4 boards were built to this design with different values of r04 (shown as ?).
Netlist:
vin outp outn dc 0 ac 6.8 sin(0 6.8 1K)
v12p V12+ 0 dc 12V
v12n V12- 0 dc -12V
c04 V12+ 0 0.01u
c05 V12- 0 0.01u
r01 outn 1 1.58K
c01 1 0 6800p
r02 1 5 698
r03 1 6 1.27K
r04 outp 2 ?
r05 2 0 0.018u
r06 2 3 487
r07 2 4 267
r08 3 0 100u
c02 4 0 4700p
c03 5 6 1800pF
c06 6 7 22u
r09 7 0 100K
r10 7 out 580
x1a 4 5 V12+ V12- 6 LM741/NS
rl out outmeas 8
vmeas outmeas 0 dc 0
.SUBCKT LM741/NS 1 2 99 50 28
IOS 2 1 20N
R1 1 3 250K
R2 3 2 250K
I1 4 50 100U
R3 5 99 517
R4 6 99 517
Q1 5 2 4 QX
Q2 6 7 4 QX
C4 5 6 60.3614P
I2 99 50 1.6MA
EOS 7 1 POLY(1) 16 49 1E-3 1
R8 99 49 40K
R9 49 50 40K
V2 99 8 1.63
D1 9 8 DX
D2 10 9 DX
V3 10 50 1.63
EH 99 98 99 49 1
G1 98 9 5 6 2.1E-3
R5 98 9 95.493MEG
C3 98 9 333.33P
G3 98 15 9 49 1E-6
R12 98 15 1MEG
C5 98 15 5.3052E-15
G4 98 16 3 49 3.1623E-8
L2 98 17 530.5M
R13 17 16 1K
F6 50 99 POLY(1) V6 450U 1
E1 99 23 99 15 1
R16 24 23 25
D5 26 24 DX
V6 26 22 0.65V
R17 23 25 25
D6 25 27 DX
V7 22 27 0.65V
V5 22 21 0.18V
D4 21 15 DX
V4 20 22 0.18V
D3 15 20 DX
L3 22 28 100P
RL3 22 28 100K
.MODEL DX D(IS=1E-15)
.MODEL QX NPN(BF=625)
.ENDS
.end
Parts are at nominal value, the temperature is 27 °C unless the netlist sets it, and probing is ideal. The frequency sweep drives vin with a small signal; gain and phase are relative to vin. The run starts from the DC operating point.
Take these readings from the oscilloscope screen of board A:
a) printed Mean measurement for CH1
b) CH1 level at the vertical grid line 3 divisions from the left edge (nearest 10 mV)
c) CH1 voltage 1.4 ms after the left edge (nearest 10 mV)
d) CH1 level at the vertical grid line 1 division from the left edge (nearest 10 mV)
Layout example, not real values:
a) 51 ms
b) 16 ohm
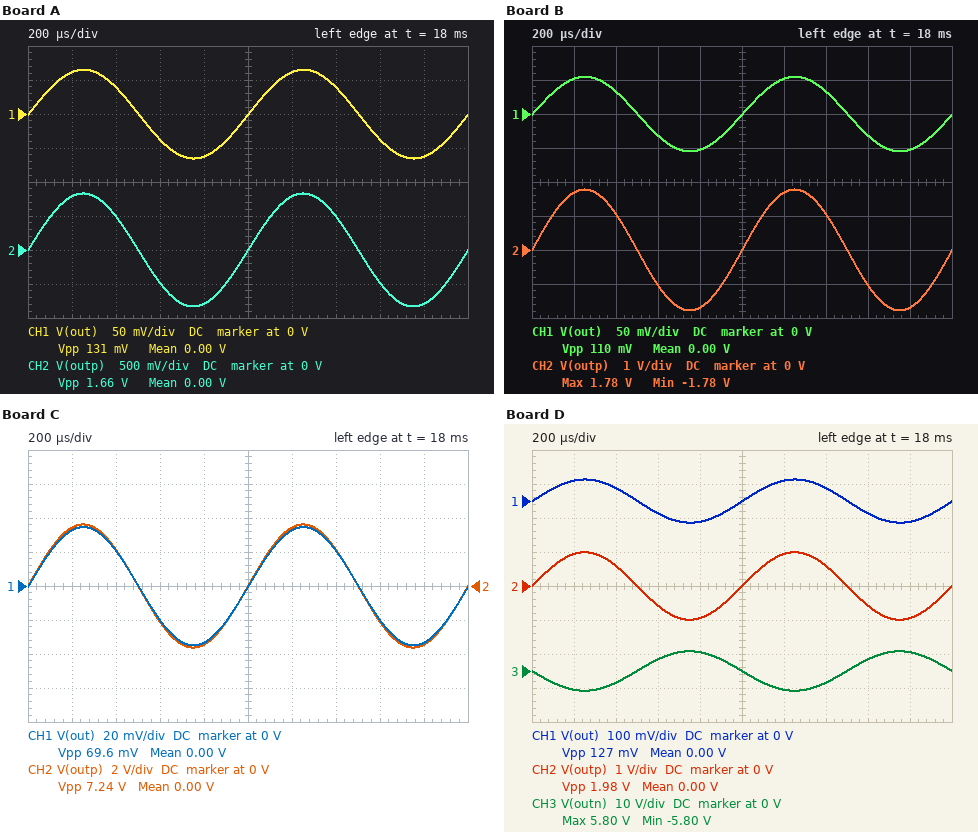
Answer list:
a) 0.00 V
b) -40 mV
c) 40 mV
d) 60 mV
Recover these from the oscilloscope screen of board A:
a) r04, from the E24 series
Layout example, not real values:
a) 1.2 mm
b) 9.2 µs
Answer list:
a) 220 Ω
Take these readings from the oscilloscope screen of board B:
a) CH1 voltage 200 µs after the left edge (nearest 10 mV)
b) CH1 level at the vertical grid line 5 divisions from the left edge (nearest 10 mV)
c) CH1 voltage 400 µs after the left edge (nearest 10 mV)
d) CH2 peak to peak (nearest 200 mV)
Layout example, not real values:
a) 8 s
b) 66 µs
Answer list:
a) 50 mV
b) 0 V
c) 30 mV
d) 3.6 V
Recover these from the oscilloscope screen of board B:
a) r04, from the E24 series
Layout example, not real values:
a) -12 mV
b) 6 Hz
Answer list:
a) 560 Ω
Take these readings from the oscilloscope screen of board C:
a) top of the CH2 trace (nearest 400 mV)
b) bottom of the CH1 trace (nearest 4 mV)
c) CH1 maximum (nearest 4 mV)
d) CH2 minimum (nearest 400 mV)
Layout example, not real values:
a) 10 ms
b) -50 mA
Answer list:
a) 3.6 V
b) -36 mV
c) 36 mV
d) -3.6 V
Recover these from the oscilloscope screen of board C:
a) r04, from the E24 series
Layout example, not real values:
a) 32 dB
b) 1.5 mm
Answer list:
a) 1.8 kΩ
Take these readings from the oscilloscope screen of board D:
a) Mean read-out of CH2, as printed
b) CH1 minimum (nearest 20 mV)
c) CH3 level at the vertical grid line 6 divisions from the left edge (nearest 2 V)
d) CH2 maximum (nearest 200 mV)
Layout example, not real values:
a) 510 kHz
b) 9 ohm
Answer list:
a) 0.00 V
b) -60 mV
c) -6 V
d) 1.0 V
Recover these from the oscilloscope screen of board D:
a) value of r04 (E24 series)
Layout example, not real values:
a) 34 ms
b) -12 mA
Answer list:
a) 270 Ω
